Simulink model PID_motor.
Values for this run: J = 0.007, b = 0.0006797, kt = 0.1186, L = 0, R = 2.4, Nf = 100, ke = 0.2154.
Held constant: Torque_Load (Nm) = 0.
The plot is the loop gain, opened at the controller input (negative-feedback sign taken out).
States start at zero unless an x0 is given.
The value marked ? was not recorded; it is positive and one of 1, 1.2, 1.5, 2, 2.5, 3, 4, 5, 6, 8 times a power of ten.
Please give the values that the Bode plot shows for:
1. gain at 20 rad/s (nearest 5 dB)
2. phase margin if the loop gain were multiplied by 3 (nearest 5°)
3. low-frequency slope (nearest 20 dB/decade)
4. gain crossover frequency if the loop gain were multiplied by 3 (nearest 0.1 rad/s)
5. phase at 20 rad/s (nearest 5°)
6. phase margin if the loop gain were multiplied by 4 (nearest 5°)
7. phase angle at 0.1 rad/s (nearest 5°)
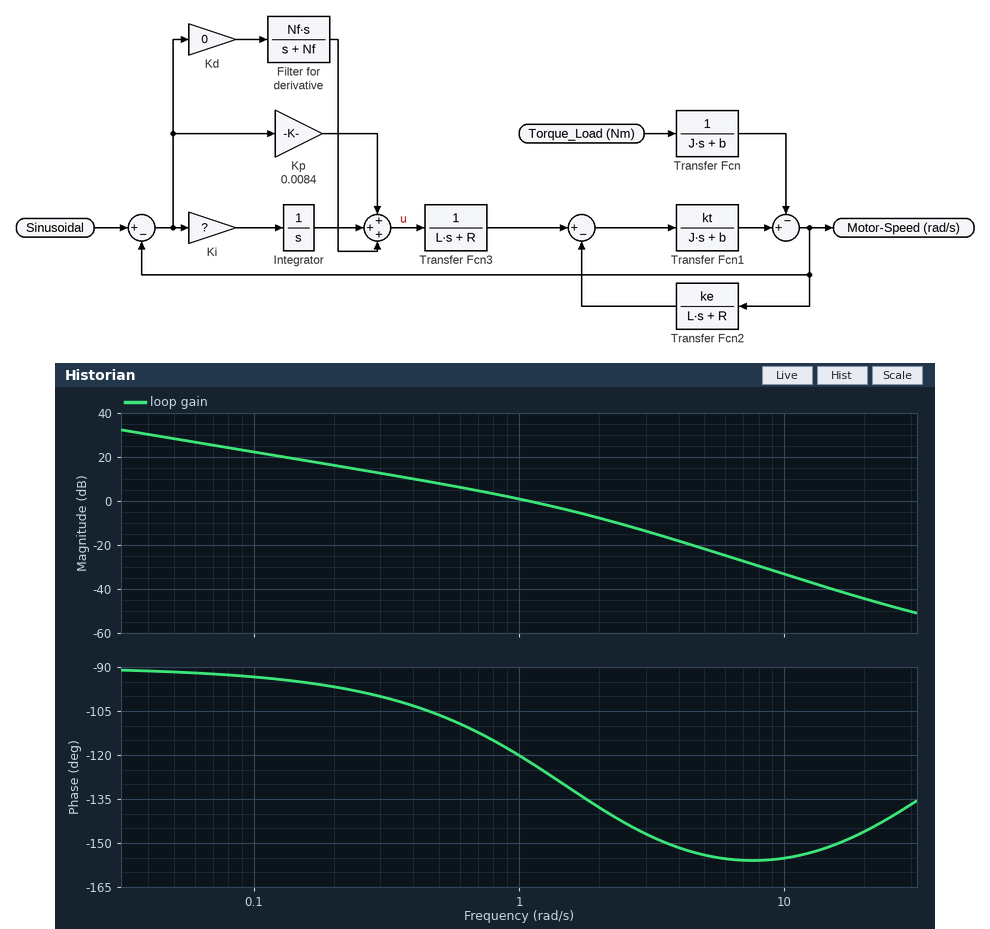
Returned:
-45 dB
40°
-20 dB/decade
2.3 rad/s
-145°
35°
-95°
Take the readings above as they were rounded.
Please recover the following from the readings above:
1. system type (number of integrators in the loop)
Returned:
1
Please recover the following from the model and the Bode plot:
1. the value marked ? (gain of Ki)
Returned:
0.3
